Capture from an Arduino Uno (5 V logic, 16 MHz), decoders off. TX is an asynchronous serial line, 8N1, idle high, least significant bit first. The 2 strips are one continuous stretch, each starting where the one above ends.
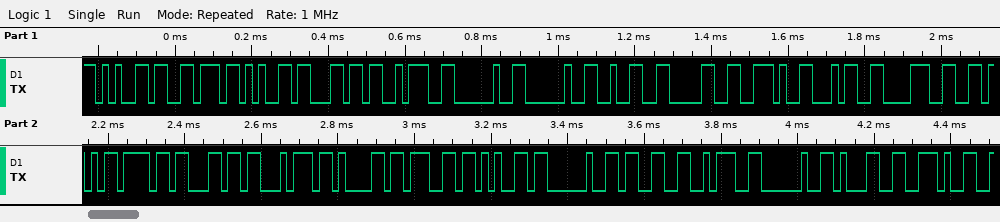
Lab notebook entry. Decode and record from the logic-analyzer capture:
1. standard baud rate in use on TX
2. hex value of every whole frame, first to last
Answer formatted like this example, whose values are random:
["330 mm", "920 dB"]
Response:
["57600 baud", "65 76 65 6C 3A 20 20 32 30 2E 34 38 56 6F 6C 74 61 67 65 20 33 3A 20 31 2E"]
